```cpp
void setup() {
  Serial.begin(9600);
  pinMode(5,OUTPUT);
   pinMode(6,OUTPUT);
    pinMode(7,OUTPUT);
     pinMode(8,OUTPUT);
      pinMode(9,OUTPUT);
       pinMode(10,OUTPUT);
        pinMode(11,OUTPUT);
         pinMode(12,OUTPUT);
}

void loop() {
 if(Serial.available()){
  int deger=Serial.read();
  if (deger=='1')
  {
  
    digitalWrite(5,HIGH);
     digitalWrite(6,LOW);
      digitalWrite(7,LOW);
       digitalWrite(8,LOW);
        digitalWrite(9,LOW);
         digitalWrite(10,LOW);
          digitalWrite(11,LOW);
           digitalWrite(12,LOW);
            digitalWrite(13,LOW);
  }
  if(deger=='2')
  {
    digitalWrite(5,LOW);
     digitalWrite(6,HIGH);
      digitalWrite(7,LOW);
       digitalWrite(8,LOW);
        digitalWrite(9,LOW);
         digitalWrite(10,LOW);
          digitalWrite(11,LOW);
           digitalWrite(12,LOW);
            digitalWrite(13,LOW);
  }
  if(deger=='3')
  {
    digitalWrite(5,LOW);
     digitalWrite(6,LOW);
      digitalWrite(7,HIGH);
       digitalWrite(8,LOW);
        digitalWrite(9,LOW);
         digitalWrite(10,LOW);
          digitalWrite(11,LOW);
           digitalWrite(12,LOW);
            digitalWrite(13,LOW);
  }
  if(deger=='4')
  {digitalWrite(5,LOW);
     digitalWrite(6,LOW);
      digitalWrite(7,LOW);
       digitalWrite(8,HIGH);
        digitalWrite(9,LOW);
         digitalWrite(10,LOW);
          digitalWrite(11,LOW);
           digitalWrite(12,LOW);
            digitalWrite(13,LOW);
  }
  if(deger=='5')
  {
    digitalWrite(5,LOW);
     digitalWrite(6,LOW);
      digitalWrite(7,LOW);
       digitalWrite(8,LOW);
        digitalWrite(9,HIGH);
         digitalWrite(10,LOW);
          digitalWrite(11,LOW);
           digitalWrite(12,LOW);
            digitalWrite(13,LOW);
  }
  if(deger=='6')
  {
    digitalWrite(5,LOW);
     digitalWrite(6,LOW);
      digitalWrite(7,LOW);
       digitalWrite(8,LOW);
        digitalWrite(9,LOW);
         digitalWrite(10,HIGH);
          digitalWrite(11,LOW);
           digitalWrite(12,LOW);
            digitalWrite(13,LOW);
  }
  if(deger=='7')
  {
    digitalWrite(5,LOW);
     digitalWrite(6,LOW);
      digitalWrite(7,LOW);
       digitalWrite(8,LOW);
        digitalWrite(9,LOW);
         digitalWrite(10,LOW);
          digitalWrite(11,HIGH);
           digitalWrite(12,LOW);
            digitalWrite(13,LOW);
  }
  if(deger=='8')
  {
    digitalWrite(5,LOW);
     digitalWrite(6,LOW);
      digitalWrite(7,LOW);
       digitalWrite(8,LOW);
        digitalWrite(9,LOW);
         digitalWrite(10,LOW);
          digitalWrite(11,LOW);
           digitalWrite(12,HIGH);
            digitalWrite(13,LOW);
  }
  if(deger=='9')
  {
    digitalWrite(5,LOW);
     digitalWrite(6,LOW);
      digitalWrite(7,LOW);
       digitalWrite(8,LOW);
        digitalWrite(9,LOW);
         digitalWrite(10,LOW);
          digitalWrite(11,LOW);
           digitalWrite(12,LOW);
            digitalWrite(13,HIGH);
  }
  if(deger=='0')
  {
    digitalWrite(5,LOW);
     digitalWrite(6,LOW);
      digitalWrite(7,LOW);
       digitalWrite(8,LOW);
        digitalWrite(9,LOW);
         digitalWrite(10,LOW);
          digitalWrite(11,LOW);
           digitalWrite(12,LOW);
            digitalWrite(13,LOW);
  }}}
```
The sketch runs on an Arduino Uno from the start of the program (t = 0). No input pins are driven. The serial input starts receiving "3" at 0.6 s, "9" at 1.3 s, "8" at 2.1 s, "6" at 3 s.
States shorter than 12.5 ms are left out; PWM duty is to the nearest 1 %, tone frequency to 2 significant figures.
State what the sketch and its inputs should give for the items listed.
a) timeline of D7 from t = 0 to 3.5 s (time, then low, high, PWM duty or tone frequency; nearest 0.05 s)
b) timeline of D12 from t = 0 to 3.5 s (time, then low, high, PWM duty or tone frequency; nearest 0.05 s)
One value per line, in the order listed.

0 s low; 0.6 s high; 1.3 s low
0 s low; 2.1 s high; 3 s low
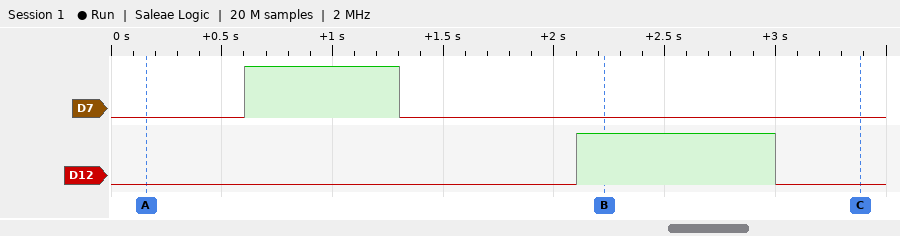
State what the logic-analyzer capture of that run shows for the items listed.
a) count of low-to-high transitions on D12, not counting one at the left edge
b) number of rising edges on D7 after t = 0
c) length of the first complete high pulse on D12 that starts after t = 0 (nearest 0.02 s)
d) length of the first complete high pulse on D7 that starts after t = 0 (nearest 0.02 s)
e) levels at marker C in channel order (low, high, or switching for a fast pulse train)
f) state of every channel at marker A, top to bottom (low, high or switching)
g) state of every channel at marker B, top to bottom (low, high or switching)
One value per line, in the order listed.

1
1
0.90 s
0.70 s
D7 low, D12 low
D7 low, D12 low
D7 low, D12 high
